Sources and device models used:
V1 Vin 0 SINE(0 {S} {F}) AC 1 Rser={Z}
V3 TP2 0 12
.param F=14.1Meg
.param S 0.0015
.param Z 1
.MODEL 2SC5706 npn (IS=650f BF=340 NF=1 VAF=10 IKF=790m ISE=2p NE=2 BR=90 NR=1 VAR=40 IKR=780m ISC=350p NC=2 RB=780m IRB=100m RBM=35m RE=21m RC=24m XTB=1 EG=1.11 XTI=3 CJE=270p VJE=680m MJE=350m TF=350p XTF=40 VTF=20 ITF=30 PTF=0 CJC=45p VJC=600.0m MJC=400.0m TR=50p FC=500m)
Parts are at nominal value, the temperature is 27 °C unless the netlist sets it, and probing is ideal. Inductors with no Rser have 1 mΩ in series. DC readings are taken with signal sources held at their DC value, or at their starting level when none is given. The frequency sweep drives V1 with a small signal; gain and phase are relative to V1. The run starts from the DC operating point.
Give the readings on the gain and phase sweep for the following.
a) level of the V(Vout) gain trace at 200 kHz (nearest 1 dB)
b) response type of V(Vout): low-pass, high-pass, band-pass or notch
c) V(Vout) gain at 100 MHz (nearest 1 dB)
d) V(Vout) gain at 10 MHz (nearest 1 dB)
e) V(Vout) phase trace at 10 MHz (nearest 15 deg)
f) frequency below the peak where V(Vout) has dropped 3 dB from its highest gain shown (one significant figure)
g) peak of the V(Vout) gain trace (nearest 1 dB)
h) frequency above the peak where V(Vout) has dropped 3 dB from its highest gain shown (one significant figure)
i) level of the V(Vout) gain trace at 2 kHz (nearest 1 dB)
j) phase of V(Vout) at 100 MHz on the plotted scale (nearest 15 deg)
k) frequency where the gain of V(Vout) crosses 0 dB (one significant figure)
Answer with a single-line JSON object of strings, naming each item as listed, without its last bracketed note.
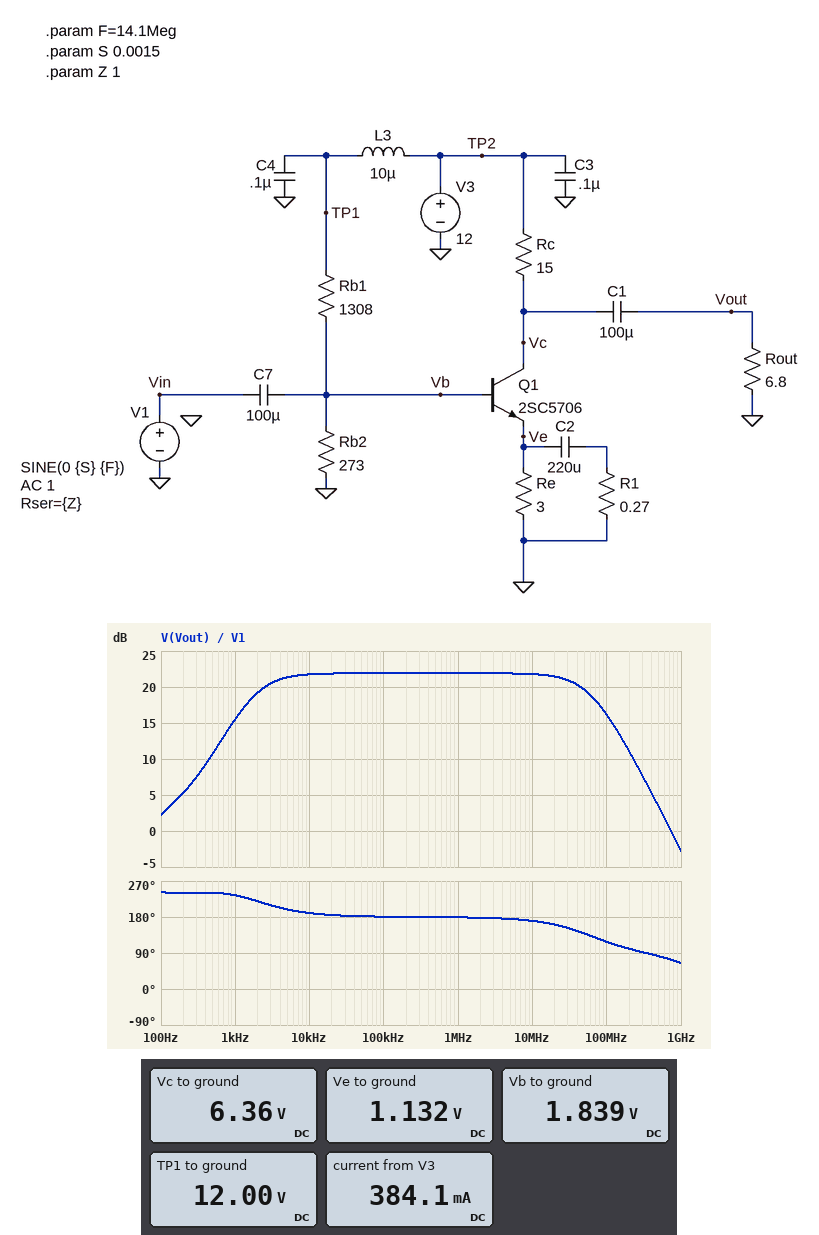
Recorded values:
{"level of the V(Vout) gain trace at 200 kHz": "22 dB", "response type of V(Vout): low-pass, high-pass, band-pass or notch": "band-pass", "V(Vout) gain at 100 MHz": "16 dB", "V(Vout) gain at 10 MHz": "22 dB", "V(Vout) phase trace at 10 MHz": "165 deg", "frequency below the peak where V(Vout) has dropped 3 dB from its highest gain shown": "2 kHz", "peak of the V(Vout) gain trace": "22 dB", "frequency above the peak where V(Vout) has dropped 3 dB from its highest gain shown": "60 MHz", "level of the V(Vout) gain trace at 2 kHz": "19 dB", "phase of V(Vout) at 100 MHz on the plotted scale": "120 deg", "frequency where the gain of V(Vout) crosses 0 dB": "700 MHz"}
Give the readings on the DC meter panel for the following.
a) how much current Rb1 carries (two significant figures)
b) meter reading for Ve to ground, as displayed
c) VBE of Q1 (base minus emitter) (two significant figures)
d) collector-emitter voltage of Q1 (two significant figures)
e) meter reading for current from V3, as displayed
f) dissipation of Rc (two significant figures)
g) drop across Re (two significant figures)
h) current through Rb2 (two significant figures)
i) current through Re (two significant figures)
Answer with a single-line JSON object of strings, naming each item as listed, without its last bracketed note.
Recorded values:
{"how much current Rb1 carries": "7.8 mA", "meter reading for Ve to ground, as displayed": "1.132 V", "VBE of Q1 (base minus emitter)": "710 mV", "collector-emitter voltage of Q1": "5.2 V", "meter reading for current from V3, as displayed": "384.1 mA", "dissipation of Rc": "2.1 W", "drop across Re": "1.1 V", "current through Rb2": "6.7 mA", "current through Re": "380 mA"}
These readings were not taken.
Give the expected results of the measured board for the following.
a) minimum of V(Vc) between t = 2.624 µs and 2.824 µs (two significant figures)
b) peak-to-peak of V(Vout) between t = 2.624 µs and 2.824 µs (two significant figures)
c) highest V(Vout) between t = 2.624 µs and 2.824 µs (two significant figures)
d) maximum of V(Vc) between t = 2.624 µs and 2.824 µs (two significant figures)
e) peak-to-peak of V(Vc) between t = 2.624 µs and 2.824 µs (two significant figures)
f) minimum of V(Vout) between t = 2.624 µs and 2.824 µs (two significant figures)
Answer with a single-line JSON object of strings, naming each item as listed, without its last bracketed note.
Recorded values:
{"minimum of V(Vc) between t = 2.624 µs and 2.824 µs": "6.3 V", "peak-to-peak of V(Vout) between t = 2.624 µs and 2.824 µs": "36 mV", "highest V(Vout) between t = 2.624 µs and 2.824 µs": "18 mV", "maximum of V(Vc) between t = 2.624 µs and 2.824 µs": "6.4 V", "peak-to-peak of V(Vc) between t = 2.624 µs and 2.824 µs": "36 mV", "minimum of V(Vout) between t = 2.624 µs and 2.824 µs": "-18 mV"}
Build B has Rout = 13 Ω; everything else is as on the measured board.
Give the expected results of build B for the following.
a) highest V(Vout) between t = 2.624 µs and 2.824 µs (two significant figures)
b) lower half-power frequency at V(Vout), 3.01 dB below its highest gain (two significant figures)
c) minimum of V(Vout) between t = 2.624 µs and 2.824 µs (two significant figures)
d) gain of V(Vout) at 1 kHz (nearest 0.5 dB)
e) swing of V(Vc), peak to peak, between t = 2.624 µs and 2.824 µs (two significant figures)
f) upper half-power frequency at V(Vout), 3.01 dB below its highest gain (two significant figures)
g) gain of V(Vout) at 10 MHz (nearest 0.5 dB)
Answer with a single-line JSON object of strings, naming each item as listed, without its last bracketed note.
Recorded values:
{"highest V(Vout) between t = 2.624 µs and 2.824 µs": "27 mV", "lower half-power frequency at V(Vout), 3.01 dB below its highest gain": "1.8 kHz", "minimum of V(Vout) between t = 2.624 µs and 2.824 µs": "-27 mV", "gain of V(Vout) at 1 kHz": "19.0 dB", "swing of V(Vc), peak to peak, between t = 2.624 µs and 2.824 µs": "53 mV", "upper half-power frequency at V(Vout), 3.01 dB below its highest gain": "56 MHz", "gain of V(Vout) at 10 MHz": "25.0 dB"}
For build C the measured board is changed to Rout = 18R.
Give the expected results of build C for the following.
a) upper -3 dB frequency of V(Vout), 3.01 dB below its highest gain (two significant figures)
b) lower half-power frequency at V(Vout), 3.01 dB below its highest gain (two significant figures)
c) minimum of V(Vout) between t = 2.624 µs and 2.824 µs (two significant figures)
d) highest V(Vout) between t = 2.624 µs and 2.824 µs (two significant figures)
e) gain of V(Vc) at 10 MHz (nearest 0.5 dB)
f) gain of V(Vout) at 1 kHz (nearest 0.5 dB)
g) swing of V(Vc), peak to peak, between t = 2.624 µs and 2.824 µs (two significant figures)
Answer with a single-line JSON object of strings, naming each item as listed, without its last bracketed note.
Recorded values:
{"upper -3 dB frequency of V(Vout), 3.01 dB below its highest gain": "54 MHz", "lower half-power frequency at V(Vout), 3.01 dB below its highest gain": "1.8 kHz", "minimum of V(Vout) between t = 2.624 µs and 2.824 µs": "-31 mV", "highest V(Vout) between t = 2.624 µs and 2.824 µs": "31 mV", "gain of V(Vc) at 10 MHz": "26.5 dB", "gain of V(Vout) at 1 kHz": "20.5 dB", "swing of V(Vc), peak to peak, between t = 2.624 µs and 2.824 µs": "62 mV"}
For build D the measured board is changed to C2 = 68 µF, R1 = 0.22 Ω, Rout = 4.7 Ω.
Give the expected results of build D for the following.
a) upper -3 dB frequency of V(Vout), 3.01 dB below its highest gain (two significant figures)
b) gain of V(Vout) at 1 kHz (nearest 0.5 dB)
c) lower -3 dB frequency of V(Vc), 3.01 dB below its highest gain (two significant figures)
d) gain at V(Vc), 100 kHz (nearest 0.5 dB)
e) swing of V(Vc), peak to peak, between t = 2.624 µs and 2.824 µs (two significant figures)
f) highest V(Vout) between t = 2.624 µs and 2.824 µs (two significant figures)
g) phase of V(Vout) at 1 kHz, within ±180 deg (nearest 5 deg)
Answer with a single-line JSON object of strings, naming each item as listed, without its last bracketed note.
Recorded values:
{"upper -3 dB frequency of V(Vout), 3.01 dB below its highest gain": "56 MHz", "gain of V(Vout) at 1 kHz": "5.5 dB", "lower -3 dB frequency of V(Vc), 3.01 dB below its highest gain": "6.9 kHz", "gain at V(Vc), 100 kHz": "20.5 dB", "swing of V(Vc), peak to peak, between t = 2.624 µs and 2.824 µs": "32 mV", "highest V(Vout) between t = 2.624 µs and 2.824 µs": "16 mV", "phase of V(Vout) at 1 kHz, within ±180 deg": "-130 deg"}
